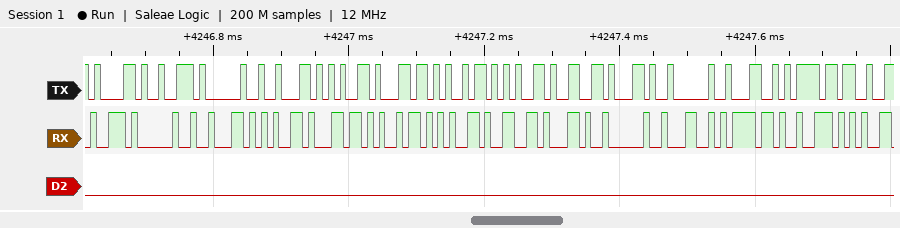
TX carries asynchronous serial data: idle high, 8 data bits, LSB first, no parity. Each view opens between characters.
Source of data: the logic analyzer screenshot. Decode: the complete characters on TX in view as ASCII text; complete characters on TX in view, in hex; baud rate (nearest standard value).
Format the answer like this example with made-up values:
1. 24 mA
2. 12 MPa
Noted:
1. "ar belief, Lo"
2. 61, 72, 20, 62, 65, 6C, 69, 65, 66, 2C, 20, 4C, 6F
3. 115200 baud
